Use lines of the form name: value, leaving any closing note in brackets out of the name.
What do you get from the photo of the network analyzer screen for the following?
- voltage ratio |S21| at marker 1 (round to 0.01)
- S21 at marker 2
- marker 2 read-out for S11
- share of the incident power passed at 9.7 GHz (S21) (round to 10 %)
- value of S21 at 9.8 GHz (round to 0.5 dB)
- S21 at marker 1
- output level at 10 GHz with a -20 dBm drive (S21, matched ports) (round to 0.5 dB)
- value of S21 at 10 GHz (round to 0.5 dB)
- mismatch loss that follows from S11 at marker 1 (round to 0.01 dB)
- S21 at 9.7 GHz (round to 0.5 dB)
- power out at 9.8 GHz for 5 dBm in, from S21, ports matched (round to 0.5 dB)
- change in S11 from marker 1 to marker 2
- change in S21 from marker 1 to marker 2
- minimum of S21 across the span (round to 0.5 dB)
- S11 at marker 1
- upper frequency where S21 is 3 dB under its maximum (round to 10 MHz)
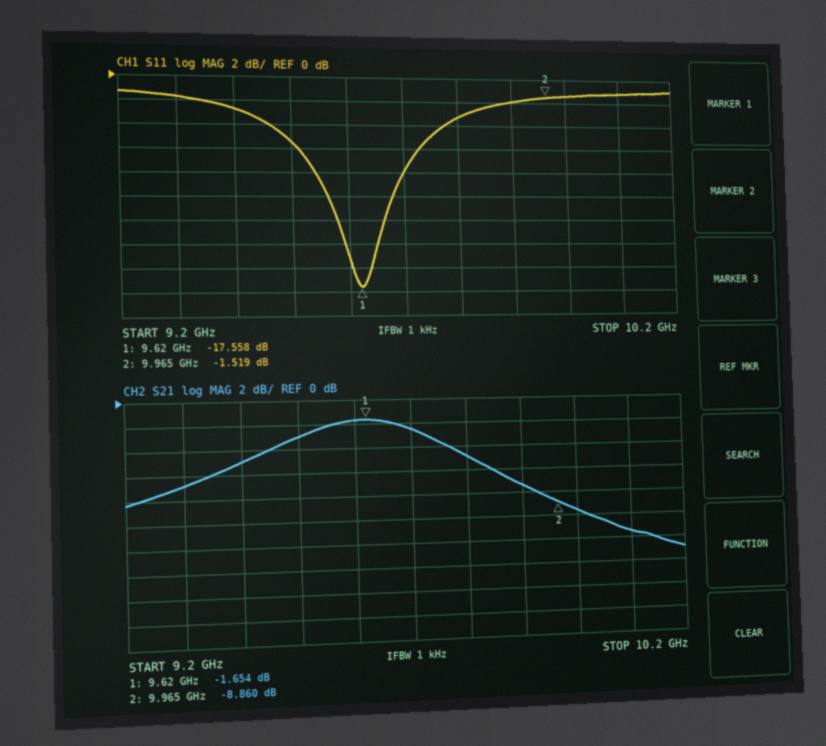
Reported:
voltage ratio |S21| at marker 1: 0.83
S21 at marker 2: -8.860 dB
marker 2 read-out for S11: -1.519 dB
share of the incident power passed at 9.7 GHz (S21): 60 %
value of S21 at 9.8 GHz: -5.0 dB
S21 at marker 1: -1.654 dB
output level at 10 GHz with a -20 dBm drive (S21, matched ports): -29.5 dBm
value of S21 at 10 GHz: -9.5 dB
mismatch loss that follows from S11 at marker 1: 0.08 dB
S21 at 9.7 GHz: -2.5 dB
power out at 9.8 GHz for 5 dBm in, from S21, ports matched: 0.0 dBm
change in S11 from marker 1 to marker 2: 16.039 dB
change in S21 from marker 1 to marker 2: -7.206 dB
minimum of S21 across the span: -13.0 dB
S11 at marker 1: -17.558 dB
upper frequency where S21 is 3 dB under its maximum: 9.79 GHz
